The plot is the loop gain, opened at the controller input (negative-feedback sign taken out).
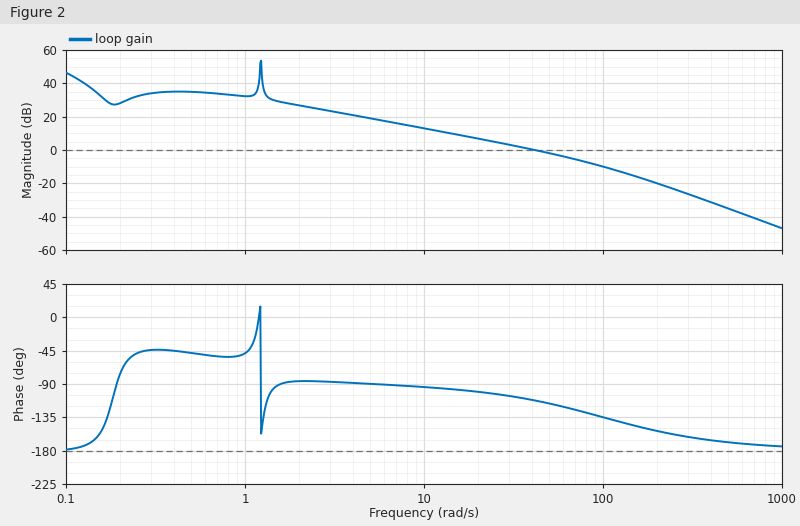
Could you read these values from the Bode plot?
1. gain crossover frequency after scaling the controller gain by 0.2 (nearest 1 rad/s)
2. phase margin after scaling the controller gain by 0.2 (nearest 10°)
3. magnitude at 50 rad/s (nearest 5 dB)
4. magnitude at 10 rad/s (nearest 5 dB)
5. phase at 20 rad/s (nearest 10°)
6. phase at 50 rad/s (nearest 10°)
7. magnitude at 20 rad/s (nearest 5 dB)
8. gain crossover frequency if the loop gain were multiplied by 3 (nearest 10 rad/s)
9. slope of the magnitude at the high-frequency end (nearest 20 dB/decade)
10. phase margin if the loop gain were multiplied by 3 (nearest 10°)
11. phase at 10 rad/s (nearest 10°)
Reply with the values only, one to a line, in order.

9 rad/s
90°
0 dB
15 dB
-100°
-120°
5 dB
100 rad/s
-40 dB/decade
50°
-90°
